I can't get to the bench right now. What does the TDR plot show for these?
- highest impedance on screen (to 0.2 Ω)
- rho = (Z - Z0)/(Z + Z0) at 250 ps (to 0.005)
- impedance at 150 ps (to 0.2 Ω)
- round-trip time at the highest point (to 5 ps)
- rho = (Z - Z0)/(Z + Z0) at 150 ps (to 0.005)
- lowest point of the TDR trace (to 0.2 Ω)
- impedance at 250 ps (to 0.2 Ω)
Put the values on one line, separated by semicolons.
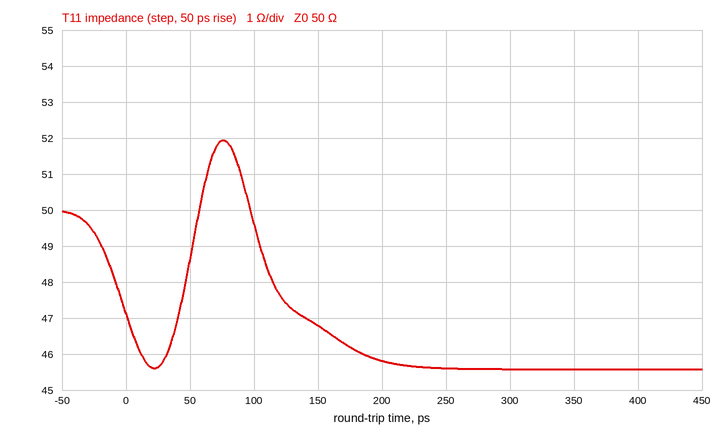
52.0 Ω; -0.045; 46.8 Ω; 75 ps; -0.035; 45.6 Ω; 45.6 Ω
